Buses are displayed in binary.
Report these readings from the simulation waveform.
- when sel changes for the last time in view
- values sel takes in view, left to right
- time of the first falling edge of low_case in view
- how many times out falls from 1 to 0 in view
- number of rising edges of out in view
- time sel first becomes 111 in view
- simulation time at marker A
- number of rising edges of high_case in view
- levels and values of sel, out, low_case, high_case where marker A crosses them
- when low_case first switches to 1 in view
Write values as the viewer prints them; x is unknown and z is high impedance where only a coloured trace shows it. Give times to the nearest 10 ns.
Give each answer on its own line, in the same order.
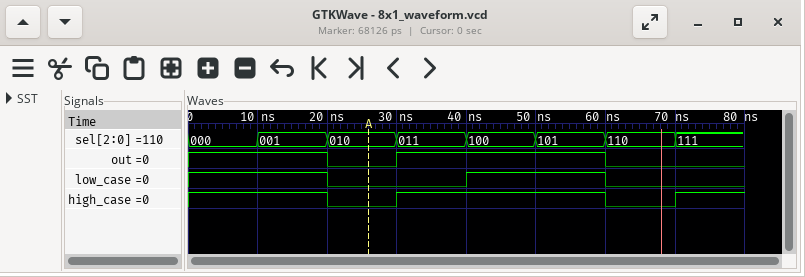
70 ns
000, 001, 010, 011, 100, 101, 110, 111
20 ns
2
1
70 ns
30 ns
2
sel=010, out=0, low_case=0, high_case=0
40 ns
